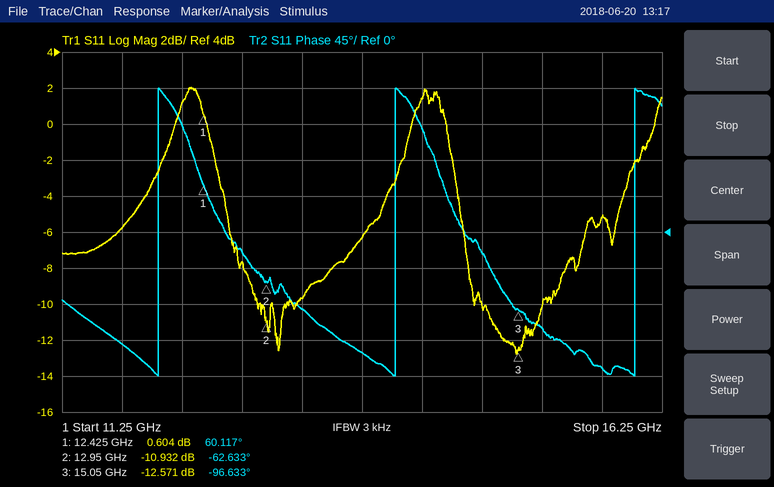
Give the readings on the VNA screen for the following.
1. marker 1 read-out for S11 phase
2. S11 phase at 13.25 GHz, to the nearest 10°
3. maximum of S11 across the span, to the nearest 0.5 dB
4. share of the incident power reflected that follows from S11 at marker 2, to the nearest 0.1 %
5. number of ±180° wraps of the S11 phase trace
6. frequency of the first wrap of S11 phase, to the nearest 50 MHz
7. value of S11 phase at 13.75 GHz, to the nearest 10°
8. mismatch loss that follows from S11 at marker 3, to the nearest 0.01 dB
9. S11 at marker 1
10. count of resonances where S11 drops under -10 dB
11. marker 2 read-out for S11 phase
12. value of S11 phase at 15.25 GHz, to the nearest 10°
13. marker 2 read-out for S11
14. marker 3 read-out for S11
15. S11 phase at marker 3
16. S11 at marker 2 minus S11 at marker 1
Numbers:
60.117°
-100°
2.0 dB
8.1 %
3
12.05 GHz
-150°
0.25 dB
0.604 dB
2
-62.633°
-120°
-10.932 dB
-12.571 dB
-96.633°
-11.536 dB
